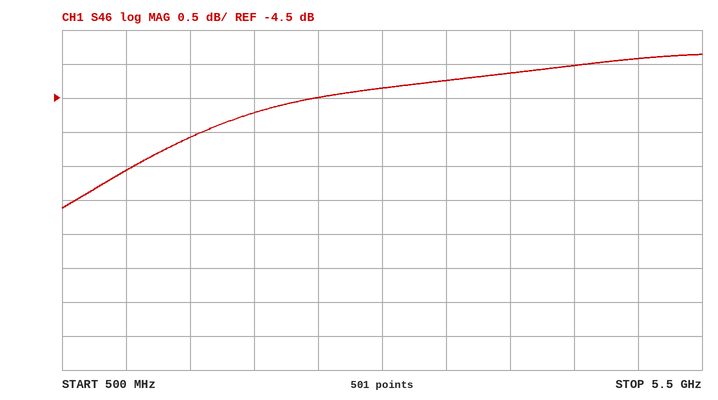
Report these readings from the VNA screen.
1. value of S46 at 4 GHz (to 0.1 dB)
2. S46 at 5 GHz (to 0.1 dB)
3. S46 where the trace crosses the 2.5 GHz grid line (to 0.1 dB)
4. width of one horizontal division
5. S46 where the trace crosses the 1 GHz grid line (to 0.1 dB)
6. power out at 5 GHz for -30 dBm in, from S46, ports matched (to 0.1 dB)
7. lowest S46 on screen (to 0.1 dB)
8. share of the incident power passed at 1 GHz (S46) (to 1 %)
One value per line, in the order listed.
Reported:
-4.1 dB
-3.9 dB
-4.5 dB
500 MHz
-5.6 dB
-33.9 dBm
-6.1 dB
28 %
